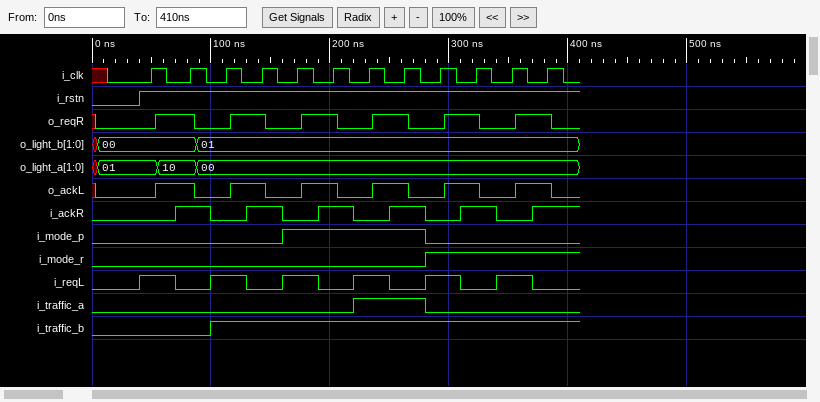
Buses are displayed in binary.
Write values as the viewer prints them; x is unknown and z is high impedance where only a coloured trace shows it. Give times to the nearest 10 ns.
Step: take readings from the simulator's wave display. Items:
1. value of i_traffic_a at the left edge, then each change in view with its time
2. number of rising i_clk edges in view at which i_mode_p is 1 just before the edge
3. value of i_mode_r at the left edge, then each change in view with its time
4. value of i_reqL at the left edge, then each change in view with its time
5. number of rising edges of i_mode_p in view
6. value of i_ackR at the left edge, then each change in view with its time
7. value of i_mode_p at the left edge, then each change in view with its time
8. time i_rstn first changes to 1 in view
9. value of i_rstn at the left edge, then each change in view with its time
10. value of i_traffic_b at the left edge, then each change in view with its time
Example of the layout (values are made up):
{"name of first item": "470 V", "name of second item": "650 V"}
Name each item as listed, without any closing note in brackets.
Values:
{"value of i_traffic_a at the left edge, then each change in view with its time": "0, 1 at 220 ns, 0 at 280 ns", "number of rising i_clk edges in view at which i_mode_p is 1 just before the edge": "4", "value of i_mode_r at the left edge, then each change in view with its time": "0, 1 at 280 ns", "value of i_reqL at the left edge, then each change in view with its time": "0, 1 at 40 ns, 0 at 70 ns, 1 at 100 ns, 0 at 130 ns, 1 at 160 ns, 0 at 190 ns, 1 at 220 ns, 0 at 250 ns, 1 at 280 ns, 0 at 310 ns, 1 at 340 ns, 0 at 370 ns", "number of rising edges of i_mode_p in view": "1", "value of i_ackR at the left edge, then each change in view with its time": "0, 1 at 70 ns, 0 at 100 ns, 1 at 130 ns, 0 at 160 ns, 1 at 190 ns, 0 at 220 ns, 1 at 250 ns, 0 at 280 ns, 1 at 310 ns, 0 at 340 ns, 1 at 370 ns", "value of i_mode_p at the left edge, then each change in view with its time": "0, 1 at 160 ns, 0 at 280 ns", "time i_rstn first changes to 1 in view": "40 ns", "value of i_rstn at the left edge, then each change in view with its time": "0, 1 at 40 ns", "value of i_traffic_b at the left edge, then each change in view with its time": "0, 1 at 100 ns"}
